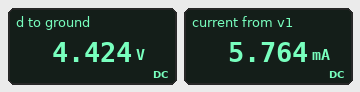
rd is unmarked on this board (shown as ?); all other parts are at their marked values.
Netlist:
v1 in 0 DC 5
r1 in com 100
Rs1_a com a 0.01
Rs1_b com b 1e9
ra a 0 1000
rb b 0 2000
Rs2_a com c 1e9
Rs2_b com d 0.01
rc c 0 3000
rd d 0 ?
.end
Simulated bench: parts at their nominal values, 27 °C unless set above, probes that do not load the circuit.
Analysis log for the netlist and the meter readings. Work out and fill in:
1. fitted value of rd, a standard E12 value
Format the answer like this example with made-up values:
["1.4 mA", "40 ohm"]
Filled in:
["3.3 kΩ"]
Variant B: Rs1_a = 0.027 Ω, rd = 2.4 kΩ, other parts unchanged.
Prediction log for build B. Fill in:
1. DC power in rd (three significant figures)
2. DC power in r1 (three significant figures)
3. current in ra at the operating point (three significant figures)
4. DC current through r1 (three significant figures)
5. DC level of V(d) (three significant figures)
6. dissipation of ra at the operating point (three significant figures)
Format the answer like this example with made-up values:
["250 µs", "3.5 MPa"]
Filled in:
["7.99 mW", "3.85 mW", "4.38 mA", "6.20 mA", "4.38 V", "19.2 mW"]
